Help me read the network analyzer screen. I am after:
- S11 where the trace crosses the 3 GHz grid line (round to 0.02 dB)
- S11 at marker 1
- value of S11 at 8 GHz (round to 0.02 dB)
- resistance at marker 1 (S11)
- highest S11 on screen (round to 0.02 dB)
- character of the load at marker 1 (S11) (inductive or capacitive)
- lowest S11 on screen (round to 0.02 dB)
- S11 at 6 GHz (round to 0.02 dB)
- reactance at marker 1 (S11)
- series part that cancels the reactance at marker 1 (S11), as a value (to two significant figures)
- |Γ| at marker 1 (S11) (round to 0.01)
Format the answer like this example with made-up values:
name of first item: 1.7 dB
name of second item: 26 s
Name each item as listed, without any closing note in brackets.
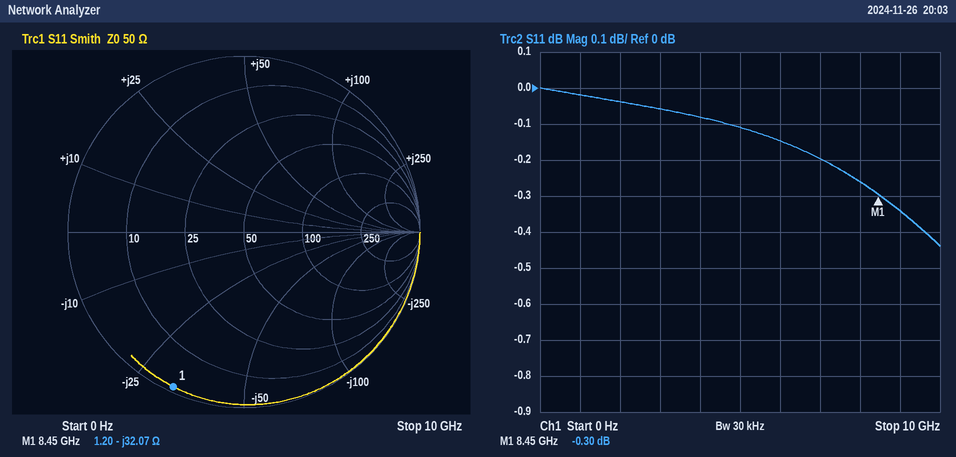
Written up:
S11 where the trace crosses the 3 GHz grid line: -0.06 dB
S11 at marker 1: -0.30 dB
value of S11 at 8 GHz: -0.26 dB
resistance at marker 1: 1.20 Ω
highest S11 on screen: 0.00 dB
character of the load at marker 1 (S11): capacitive
lowest S11 on screen: -0.44 dB
S11 at 6 GHz: -0.14 dB
reactance at marker 1: -32.07 Ω
series part that cancels the reactance at marker 1 (S11), as a value: 600 pH
|Γ| at marker 1 (S11): 0.97
